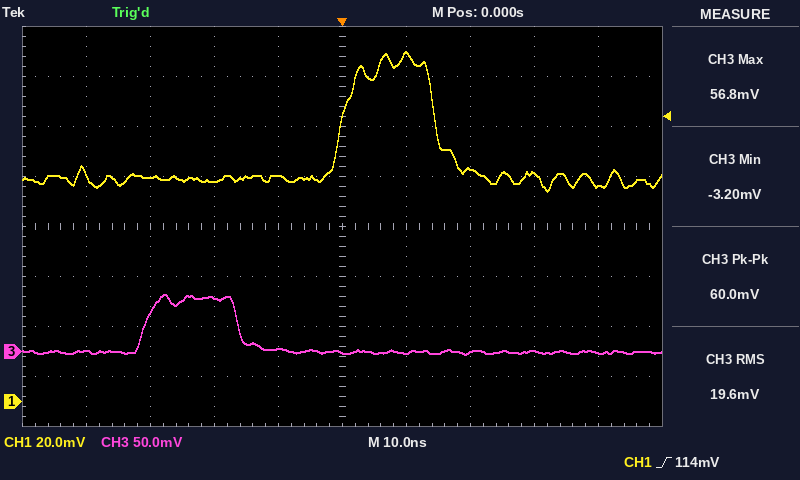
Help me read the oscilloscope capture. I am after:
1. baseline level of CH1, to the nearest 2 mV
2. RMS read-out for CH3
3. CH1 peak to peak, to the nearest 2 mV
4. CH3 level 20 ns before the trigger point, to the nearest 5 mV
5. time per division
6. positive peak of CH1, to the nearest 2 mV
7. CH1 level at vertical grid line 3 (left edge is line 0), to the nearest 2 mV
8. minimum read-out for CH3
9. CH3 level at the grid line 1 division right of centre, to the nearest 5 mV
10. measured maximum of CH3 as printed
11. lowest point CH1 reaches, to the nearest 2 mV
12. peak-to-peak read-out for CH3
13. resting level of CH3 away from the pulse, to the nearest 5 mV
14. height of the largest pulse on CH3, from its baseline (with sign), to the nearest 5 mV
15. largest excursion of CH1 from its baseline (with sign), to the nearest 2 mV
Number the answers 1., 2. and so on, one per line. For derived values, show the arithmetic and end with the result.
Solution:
1. 90 mV
2. 19.6 mV
3. 140 mV − (84 mV) = 56 mV
4. 55 mV
5. 10 ns
6. 140 mV
7. 88 mV
8. -3.20 mV
9. 0 mV
10. 56.8 mV
11. 84 mV
12. 60.0 mV
13. 0 mV
14. +55 mV
15. 140 mV − (90 mV) = +50 mV
